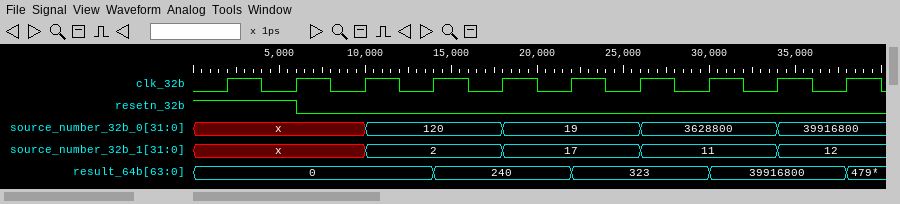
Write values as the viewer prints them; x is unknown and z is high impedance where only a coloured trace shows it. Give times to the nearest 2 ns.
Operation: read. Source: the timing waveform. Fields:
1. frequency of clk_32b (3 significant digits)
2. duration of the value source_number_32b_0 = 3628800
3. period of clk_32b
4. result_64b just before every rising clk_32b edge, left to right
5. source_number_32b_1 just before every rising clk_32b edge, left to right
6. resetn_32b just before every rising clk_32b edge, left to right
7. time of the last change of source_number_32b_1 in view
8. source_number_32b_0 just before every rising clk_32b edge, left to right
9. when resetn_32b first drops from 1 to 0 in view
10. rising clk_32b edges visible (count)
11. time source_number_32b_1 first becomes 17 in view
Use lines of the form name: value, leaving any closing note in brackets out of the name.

frequency of clk_32b: 250 MHz
duration of the value source_number_32b_0 = 3628800: 8 ns
period of clk_32b: 4 ns
result_64b just before every rising clk_32b edge, left to right: 0, 0, 0, 0, 240, 240, 323, 323, 39916800, 39916800
source_number_32b_1 just before every rising clk_32b edge, left to right: x, x, x, 2, 2, 17, 17, 11, 11, 12
resetn_32b just before every rising clk_32b edge, left to right: 1 1 0 0 0 0 0 0 0 0
time of the last change of source_number_32b_1 in view: 34 ns
source_number_32b_0 just before every rising clk_32b edge, left to right: x, x, x, 120, 120, 19, 19, 3628800, 3628800, 39916800
when resetn_32b first drops from 1 to 0 in view: 6 ns
rising clk_32b edges visible: 10
time source_number_32b_1 first becomes 17 in view: 18 ns
